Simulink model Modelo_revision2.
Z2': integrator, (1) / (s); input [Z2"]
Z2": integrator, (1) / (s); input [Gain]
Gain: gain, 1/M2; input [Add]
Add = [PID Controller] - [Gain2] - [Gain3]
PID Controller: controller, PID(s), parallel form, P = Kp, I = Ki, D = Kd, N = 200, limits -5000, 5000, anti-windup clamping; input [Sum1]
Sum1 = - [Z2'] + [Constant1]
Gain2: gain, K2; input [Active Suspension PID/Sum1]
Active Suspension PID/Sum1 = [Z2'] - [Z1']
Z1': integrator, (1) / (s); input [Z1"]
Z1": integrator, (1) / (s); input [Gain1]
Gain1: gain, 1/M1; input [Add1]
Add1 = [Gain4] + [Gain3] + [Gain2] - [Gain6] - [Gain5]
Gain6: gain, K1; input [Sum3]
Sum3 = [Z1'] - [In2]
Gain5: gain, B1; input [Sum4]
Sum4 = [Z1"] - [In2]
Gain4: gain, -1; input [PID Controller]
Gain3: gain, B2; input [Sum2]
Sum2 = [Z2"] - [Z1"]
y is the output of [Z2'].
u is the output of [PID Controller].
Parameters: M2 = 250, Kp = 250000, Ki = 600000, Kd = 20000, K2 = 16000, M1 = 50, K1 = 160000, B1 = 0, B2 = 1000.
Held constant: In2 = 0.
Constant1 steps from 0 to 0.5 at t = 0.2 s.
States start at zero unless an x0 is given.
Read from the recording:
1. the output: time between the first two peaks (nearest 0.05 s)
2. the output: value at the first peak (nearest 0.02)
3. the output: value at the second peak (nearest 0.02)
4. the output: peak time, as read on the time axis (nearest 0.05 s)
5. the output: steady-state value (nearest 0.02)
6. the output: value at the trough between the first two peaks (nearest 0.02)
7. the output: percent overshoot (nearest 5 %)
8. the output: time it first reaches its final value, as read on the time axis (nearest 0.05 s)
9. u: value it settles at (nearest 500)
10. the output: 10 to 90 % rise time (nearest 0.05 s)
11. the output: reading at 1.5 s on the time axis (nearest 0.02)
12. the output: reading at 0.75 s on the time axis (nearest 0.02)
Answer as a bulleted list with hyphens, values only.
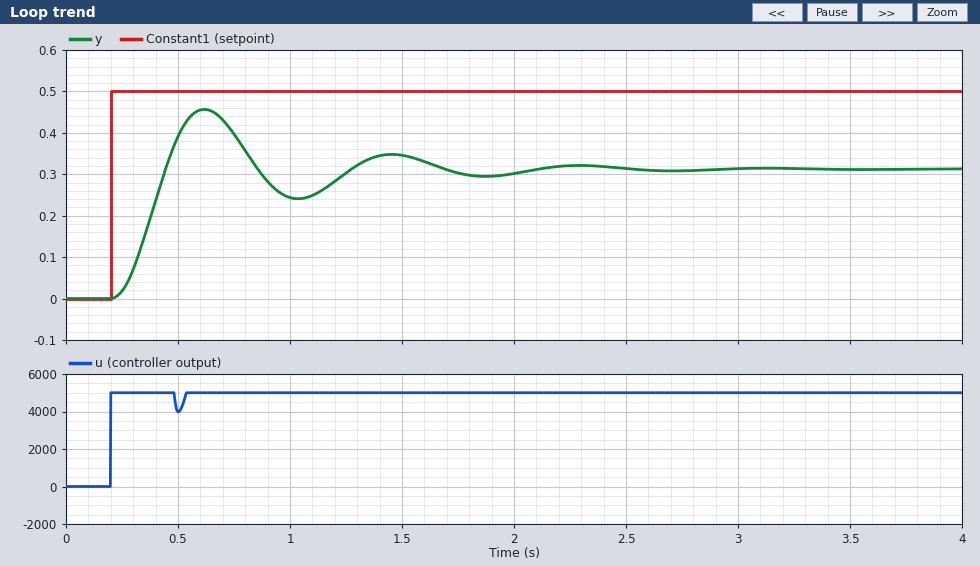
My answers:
- 0.85 s
- 0.46
- 0.34
- 0.60 s
- 0.32
- 0.24
- 45 %
- 0.45 s
- 5000
- 0.15 s
- 0.34
- 0.40
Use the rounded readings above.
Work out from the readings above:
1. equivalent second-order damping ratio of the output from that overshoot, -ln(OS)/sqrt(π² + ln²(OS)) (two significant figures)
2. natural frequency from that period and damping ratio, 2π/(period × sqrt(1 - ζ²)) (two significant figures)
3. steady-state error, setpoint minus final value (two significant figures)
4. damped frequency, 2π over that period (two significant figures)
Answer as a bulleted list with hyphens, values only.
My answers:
- 0.25
- 7.6 rad/s
- 0.18
- 7.4 rad/s
